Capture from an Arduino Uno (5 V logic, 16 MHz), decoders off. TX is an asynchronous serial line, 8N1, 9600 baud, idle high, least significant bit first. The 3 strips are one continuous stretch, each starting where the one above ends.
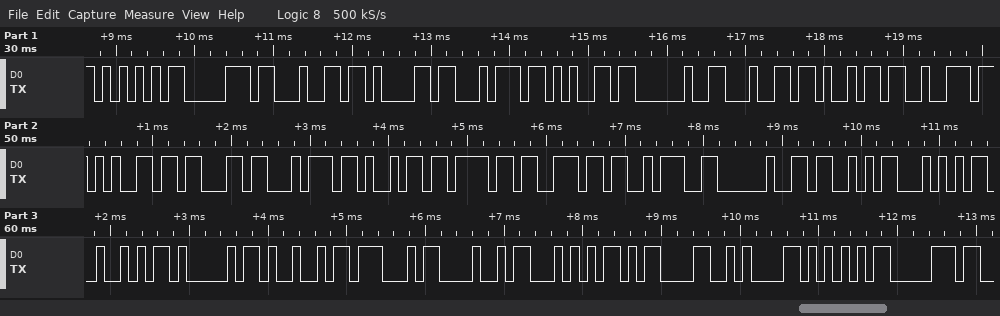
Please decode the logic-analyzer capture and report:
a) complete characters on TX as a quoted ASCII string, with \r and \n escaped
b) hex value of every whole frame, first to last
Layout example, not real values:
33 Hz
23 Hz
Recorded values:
"Update direction: STRAIGHT\r\nUp"
55 70 64 61 74 65 20 64 69 72 65 63 74 69 6F 6E 3A 20 53 54 52 41 49 47 48 54 0D 0A 55 70
